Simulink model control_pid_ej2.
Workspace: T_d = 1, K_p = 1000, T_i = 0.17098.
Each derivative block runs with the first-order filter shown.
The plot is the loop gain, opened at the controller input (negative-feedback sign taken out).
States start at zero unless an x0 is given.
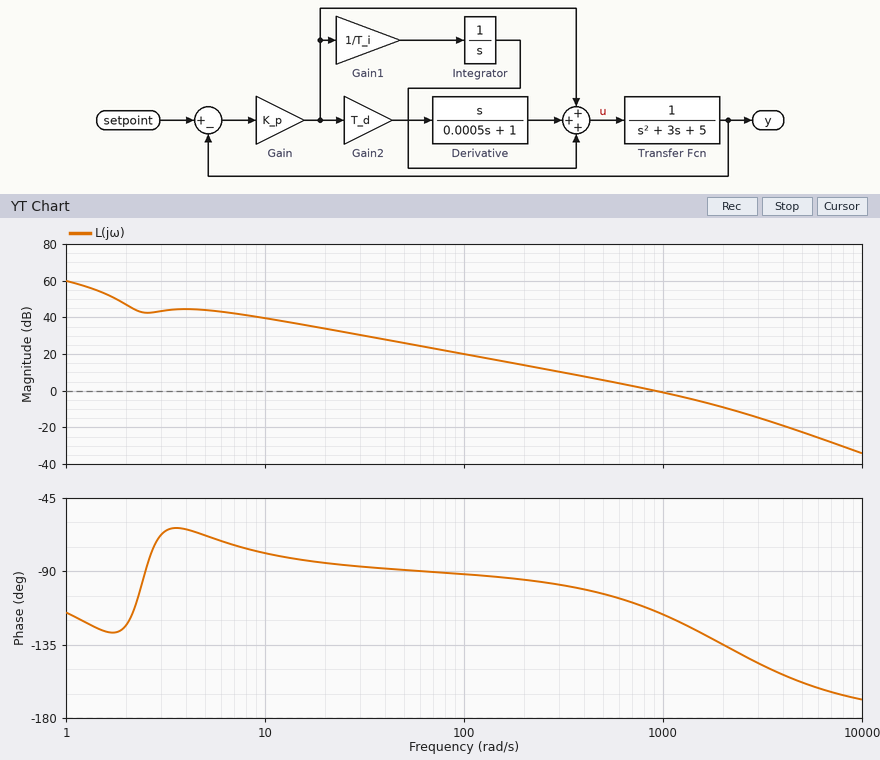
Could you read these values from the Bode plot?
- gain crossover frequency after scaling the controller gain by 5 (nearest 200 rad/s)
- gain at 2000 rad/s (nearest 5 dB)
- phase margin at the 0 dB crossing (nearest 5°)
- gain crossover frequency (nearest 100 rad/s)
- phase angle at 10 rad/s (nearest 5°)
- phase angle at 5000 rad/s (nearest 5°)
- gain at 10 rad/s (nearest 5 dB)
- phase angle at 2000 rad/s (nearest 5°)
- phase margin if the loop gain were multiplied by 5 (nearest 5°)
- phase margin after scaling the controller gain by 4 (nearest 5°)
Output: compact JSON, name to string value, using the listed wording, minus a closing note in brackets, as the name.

{"gain crossover frequency after scaling the controller gain by 5": "2800 rad/s", "gain at 2000 rad/s": "-10 dB", "phase margin at the 0 dB crossing": "65°", "gain crossover frequency": "900 rad/s", "phase angle at 10 rad/s": "-80°", "phase angle at 5000 rad/s": "-160°", "gain at 10 rad/s": "40 dB", "phase angle at 2000 rad/s": "-135°", "phase margin if the loop gain were multiplied by 5": "35°", "phase margin after scaling the controller gain by 4": "40°"}
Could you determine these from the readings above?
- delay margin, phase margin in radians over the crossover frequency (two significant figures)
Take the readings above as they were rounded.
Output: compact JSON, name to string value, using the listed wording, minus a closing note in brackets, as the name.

{"delay margin, phase margin in radians over the crossover frequency": "0.0013 s"}
